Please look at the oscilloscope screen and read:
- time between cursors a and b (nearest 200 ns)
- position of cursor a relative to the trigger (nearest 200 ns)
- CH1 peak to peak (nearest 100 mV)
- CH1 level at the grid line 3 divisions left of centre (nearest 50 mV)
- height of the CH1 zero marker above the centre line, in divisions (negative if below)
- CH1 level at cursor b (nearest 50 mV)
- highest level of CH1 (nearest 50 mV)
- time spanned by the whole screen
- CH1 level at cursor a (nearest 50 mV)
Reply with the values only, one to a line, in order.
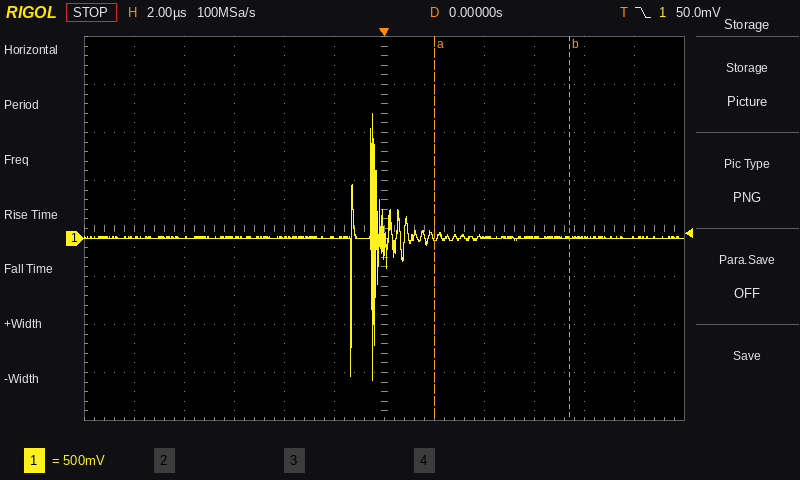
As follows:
5.4 µs
+2.0 µs
2.80 V
0 mV
-0.2 div
0 mV
1.30 V
24 µs
0 mV
